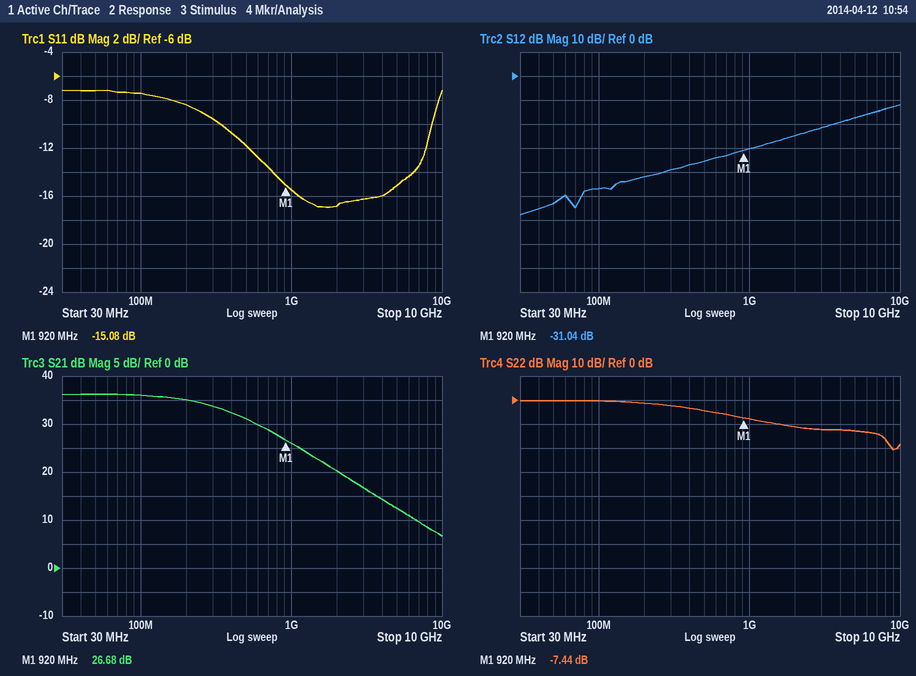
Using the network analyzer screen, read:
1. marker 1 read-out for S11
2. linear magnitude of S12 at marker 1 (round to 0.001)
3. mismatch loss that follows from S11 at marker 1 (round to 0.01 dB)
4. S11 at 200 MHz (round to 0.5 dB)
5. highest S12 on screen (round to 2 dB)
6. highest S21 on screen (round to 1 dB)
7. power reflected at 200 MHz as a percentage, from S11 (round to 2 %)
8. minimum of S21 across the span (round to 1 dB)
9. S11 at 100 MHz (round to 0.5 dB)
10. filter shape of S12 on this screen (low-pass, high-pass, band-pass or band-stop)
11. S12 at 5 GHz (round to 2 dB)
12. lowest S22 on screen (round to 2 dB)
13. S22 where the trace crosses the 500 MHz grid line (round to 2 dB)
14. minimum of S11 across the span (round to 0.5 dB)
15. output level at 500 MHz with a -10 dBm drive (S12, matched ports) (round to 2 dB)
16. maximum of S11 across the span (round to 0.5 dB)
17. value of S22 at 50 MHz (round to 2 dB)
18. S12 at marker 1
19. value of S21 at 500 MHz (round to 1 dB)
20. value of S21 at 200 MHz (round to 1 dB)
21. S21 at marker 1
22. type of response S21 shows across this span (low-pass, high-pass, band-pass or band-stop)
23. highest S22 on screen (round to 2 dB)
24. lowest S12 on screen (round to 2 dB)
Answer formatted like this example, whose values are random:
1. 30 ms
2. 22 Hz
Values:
1. -15.08 dB
2. 0.028
3. 0.14 dB
4. -8.5 dB
5. -12 dB
6. 36 dB
7. 14 %
8. 7 dB
9. -7.5 dB
10. high-pass
11. -18 dB
12. -20 dB
13. -4 dB
14. -17.0 dB
15. -46 dBm
16. -7.0 dB
17. 0 dB
18. -31.04 dB
19. 31 dB
20. 35 dB
21. 26.68 dB
22. low-pass
23. 0 dB
24. -58 dB
